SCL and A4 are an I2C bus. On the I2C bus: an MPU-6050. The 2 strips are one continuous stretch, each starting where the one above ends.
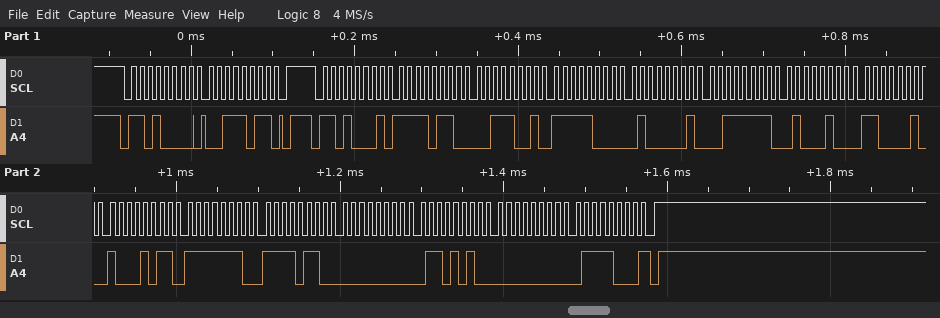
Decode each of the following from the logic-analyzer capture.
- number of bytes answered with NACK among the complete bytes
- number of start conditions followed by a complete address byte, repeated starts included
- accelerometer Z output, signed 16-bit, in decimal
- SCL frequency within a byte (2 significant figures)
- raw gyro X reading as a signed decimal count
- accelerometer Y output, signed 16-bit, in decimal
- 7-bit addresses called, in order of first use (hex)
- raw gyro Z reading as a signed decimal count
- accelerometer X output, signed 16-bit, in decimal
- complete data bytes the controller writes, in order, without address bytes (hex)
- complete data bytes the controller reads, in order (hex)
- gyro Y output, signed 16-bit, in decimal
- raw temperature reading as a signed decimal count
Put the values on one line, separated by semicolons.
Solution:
1; 2; 16196; 100 kHz; -266; -1983; 0x68; 120; -2503; 3B; F6 39 F8 41 3F 44 C2 8B FE F6 00 6A 00 78; 106; -15733
